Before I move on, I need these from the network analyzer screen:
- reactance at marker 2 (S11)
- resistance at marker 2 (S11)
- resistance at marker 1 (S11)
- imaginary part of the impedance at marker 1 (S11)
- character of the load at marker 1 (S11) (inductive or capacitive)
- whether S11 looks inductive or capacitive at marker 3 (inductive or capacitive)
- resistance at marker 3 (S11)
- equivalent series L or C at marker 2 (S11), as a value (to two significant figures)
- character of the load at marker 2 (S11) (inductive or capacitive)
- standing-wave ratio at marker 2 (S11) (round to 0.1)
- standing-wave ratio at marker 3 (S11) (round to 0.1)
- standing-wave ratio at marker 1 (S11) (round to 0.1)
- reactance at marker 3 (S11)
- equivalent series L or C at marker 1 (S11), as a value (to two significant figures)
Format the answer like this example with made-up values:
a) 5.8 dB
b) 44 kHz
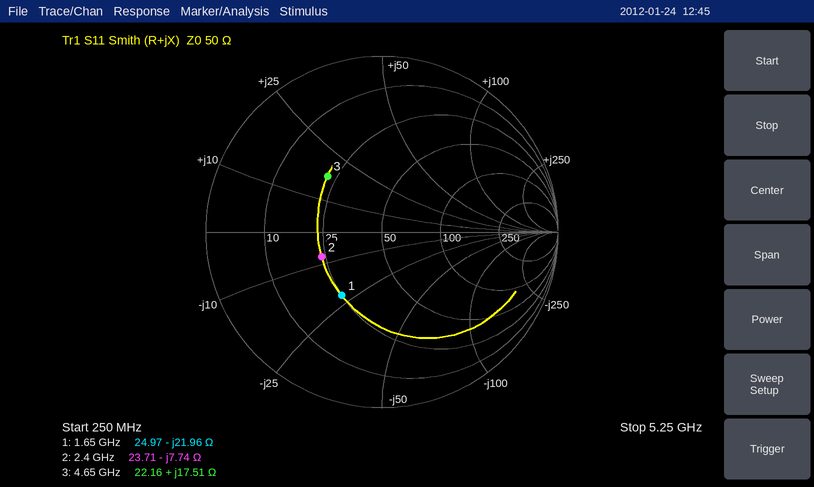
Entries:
a) -7.74 Ω
b) 23.71 Ω
c) 24.97 Ω
d) -21.96 Ω
e) capacitive
f) inductive
g) 22.16 Ω
h) 8.6 pF
i) capacitive
j) 2.2
k) 2.6
l) 2.5
m) +17.51 Ω
n) 4.4 pF
